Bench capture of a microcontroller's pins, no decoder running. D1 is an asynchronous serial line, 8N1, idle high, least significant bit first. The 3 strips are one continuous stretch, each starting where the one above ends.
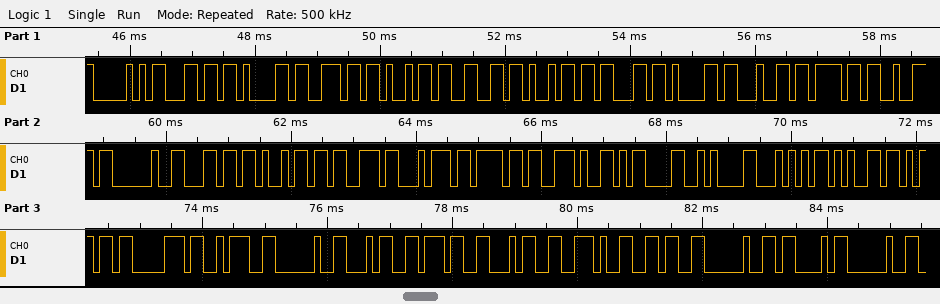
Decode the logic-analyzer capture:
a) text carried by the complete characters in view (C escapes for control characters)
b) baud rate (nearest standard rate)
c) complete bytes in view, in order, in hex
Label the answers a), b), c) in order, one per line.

a) "Planificador listo.\r\nTemp: 474.6 C "
b) 9600 baud
c) 50 6C 61 6E 69 66 69 63 61 64 6F 72 20 6C 69 73 74 6F 2E 0D 0A 54 65 6D 70 3A 20 34 37 34 2E 36 20 43 20
